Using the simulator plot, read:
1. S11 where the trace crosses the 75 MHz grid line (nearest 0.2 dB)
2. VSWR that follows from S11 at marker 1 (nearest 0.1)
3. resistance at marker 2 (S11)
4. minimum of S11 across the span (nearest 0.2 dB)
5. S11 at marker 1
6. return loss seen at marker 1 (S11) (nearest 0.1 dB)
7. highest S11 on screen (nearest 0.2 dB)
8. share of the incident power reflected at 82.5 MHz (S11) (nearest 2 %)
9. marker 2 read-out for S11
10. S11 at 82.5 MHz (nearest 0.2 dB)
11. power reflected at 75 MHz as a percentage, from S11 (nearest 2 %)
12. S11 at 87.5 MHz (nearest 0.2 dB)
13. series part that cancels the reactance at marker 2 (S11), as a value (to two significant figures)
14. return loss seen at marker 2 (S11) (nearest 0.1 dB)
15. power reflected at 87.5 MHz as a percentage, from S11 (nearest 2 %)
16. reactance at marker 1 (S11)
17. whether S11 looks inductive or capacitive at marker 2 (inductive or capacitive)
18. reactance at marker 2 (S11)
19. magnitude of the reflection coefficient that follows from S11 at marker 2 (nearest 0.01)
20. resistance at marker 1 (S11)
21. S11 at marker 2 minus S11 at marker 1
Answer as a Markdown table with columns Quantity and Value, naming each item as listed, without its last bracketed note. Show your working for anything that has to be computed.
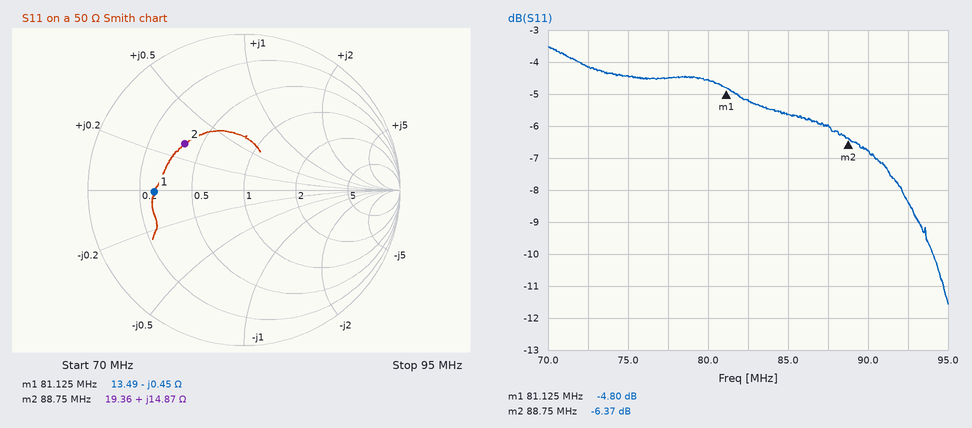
| Quantity | Value |
|---|---|
| S11 where the trace crosses the 75 MHz grid line | -4.4 dB |
| VSWR that follows from S11 at marker 1 | (1 + 0.5754)/(1 − 0.5754) ≈ 3.7 |
| resistance at marker 2 | 19.36 Ω |
| minimum of S11 across the span | -11.6 dB |
| S11 at marker 1 | -4.80 dB |
| return loss seen at marker 1 (S11) | 4.8 dB |
| highest S11 on screen | -3.6 dB |
| share of the incident power reflected at 82.5 MHz (S11) | 10^(-5.2/10) ≈ 30 % |
| marker 2 read-out for S11 | -6.37 dB |
| S11 at 82.5 MHz | -5.2 dB |
| power reflected at 75 MHz as a percentage, from S11 | 10^(-4.4/10) ≈ 36 % |
| S11 at 87.5 MHz | -6.0 dB |
| series part that cancels the reactance at marker 2 (S11), as a value | C = 1/(2π × 88.75 MHz × 14.87 Ω) ≈ 121 pF, so 120 pF to two significant figures |
| return loss seen at marker 2 (S11) | 6.4 dB |
| power reflected at 87.5 MHz as a percentage, from S11 | 10^(-6/10) ≈ 25.1 %, so 26 % to the nearest 2 % |
| reactance at marker 1 | -0.45 Ω |
| whether S11 looks inductive or capacitive at marker 2 | inductive |
| reactance at marker 2 | +14.87 Ω |
| magnitude of the reflection coefficient that follows from S11 at marker 2 | 10^(-6.37/20) ≈ 0.48 |
| resistance at marker 1 | 13.49 Ω |
| S11 at marker 2 minus S11 at marker 1 | -6.37 − (-4.8) = -1.57 dB |
